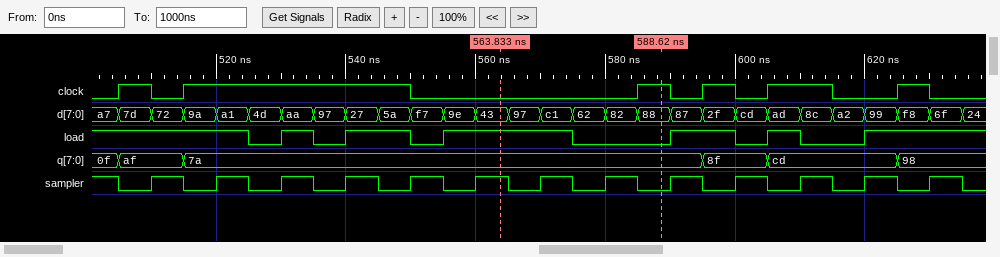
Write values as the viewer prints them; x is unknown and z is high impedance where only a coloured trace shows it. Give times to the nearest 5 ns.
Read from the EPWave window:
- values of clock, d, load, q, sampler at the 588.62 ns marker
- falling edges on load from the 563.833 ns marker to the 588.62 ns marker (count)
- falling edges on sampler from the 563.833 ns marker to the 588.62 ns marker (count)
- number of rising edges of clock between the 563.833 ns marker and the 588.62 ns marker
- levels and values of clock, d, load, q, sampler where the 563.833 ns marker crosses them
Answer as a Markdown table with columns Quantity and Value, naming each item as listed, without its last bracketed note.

| Quantity | Value |
|---|---|
| values of clock, d, load, q, sampler at the 588.62 ns marker | clock=1, d=88, load=0, q=7a, sampler=0 |
| falling edges on load from the 563.833 ns marker to the 588.62 ns marker | 1 |
| falling edges on sampler from the 563.833 ns marker to the 588.62 ns marker | 3 |
| number of rising edges of clock between the 563.833 ns marker and the 588.62 ns marker | 1 |
| levels and values of clock, d, load, q, sampler where the 563.833 ns marker crosses them | clock=0, d=43, load=1, q=7a, sampler=1 |
